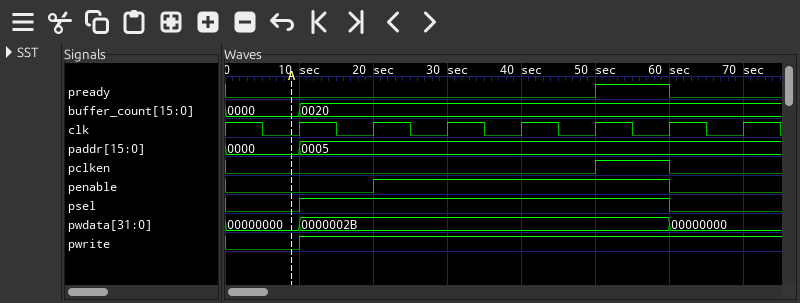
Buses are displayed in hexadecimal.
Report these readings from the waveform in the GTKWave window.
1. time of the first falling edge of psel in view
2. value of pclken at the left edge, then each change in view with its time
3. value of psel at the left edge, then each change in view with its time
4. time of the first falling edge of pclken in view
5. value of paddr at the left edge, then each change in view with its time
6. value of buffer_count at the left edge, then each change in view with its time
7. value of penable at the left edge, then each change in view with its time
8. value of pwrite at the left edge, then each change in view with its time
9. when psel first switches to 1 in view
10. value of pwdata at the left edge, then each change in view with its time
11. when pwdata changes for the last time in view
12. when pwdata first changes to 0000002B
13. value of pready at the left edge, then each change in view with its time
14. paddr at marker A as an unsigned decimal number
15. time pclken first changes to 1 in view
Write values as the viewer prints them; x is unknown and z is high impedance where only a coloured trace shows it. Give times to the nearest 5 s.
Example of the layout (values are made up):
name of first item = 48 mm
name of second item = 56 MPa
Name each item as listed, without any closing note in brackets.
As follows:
time of the first falling edge of psel in view = 60 s
value of pclken at the left edge, then each change in view with its time = 0, 1 at 50 s, 0 at 60 s
value of psel at the left edge, then each change in view with its time = 0, 1 at 10 s, 0 at 60 s
time of the first falling edge of pclken in view = 60 s
value of paddr at the left edge, then each change in view with its time = 0000, 0005 at 10 s
value of buffer_count at the left edge, then each change in view with its time = 0000, 0020 at 10 s
value of penable at the left edge, then each change in view with its time = 0, 1 at 20 s, 0 at 60 s
value of pwrite at the left edge, then each change in view with its time = 0, 1 at 10 s
when psel first switches to 1 in view = 10 s
value of pwdata at the left edge, then each change in view with its time = 00000000, 0000002B at 10 s, 00000000 at 60 s
when pwdata changes for the last time in view = 60 s
when pwdata first changes to 0000002B = 10 s
value of pready at the left edge, then each change in view with its time = 0, 1 at 50 s, 0 at 60 s
paddr at marker A as an unsigned decimal number = 0
time pclken first changes to 1 in view = 50 s
